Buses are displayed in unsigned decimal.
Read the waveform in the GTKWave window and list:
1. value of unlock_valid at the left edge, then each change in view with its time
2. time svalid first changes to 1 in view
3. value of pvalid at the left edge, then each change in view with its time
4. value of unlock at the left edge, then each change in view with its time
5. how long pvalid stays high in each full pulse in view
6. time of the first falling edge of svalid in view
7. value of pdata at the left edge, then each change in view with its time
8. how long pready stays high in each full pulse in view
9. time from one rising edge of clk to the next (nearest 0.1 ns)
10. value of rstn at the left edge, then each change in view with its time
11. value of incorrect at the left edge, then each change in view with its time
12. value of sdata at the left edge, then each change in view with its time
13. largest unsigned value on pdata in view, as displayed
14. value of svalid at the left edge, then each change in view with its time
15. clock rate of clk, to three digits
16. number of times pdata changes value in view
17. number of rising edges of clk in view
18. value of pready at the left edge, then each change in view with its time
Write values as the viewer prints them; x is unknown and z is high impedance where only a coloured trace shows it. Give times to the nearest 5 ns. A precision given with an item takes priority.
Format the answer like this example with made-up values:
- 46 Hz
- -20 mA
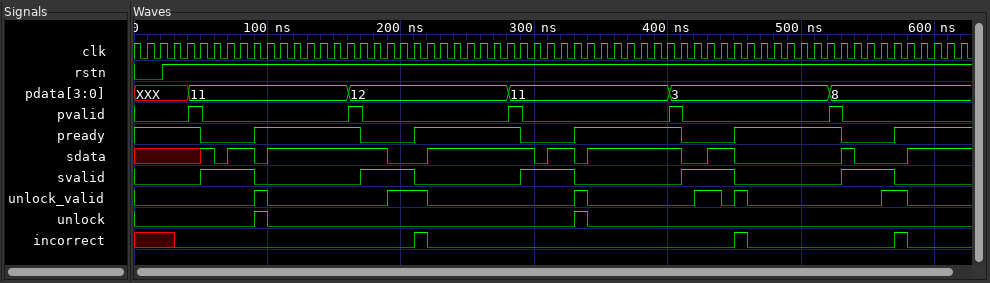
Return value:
- 0, 1 at 90 ns, 0 at 100 ns, 1 at 190 ns, 0 at 220 ns, 1 at 330 ns, 0 at 340 ns, 1 at 420 ns, 0 at 440 ns, 1 at 450 ns, 0 at 460 ns, 1 at 560 ns, 0 at 580 ns
- 50 ns
- 0, 1 at 40 ns, 0 at 50 ns, 1 at 160 ns, 0 at 170 ns, 1 at 280 ns, 0 at 290 ns, 1 at 400 ns, 0 at 410 ns, 1 at 520 ns, 0 at 530 ns
- 0, 1 at 90 ns, 0 at 100 ns, 1 at 330 ns, 0 at 340 ns
- 10 ns, 10 ns, 10 ns, 10 ns, 10 ns
- 90 ns
- XXX, 11 at 40 ns, 12 at 160 ns, 11 at 280 ns, 3 at 400 ns, 8 at 520 ns
- 80 ns, 80 ns, 80 ns, 80 ns
- 10 ns
- 0, 1 at 20 ns
- x, 0 at 30 ns, 1 at 210 ns, 0 at 220 ns, 1 at 450 ns, 0 at 460 ns, 1 at 570 ns, 0 at 580 ns
- x, 1 at 50 ns, 0 at 60 ns, 1 at 70 ns, 0 at 90 ns, 1 at 100 ns, 0 at 190 ns, 1 at 220 ns, 0 at 300 ns, 1 at 310 ns, 0 at 330 ns, 1 at 340 ns, 0 at 410 ns, 1 at 430 ns, 0 at 450 ns, 1 at 530 ns, 0 at 540 ns, 1 at 580 ns
- 12
- 0, 1 at 50 ns, 0 at 90 ns, 1 at 170 ns, 0 at 210 ns, 1 at 290 ns, 0 at 330 ns, 1 at 410 ns, 0 at 450 ns, 1 at 530 ns, 0 at 570 ns
- 100 MHz
- 5
- 62
- 1, 0 at 50 ns, 1 at 90 ns, 0 at 170 ns, 1 at 210 ns, 0 at 290 ns, 1 at 330 ns, 0 at 410 ns, 1 at 450 ns, 0 at 530 ns, 1 at 570 ns
